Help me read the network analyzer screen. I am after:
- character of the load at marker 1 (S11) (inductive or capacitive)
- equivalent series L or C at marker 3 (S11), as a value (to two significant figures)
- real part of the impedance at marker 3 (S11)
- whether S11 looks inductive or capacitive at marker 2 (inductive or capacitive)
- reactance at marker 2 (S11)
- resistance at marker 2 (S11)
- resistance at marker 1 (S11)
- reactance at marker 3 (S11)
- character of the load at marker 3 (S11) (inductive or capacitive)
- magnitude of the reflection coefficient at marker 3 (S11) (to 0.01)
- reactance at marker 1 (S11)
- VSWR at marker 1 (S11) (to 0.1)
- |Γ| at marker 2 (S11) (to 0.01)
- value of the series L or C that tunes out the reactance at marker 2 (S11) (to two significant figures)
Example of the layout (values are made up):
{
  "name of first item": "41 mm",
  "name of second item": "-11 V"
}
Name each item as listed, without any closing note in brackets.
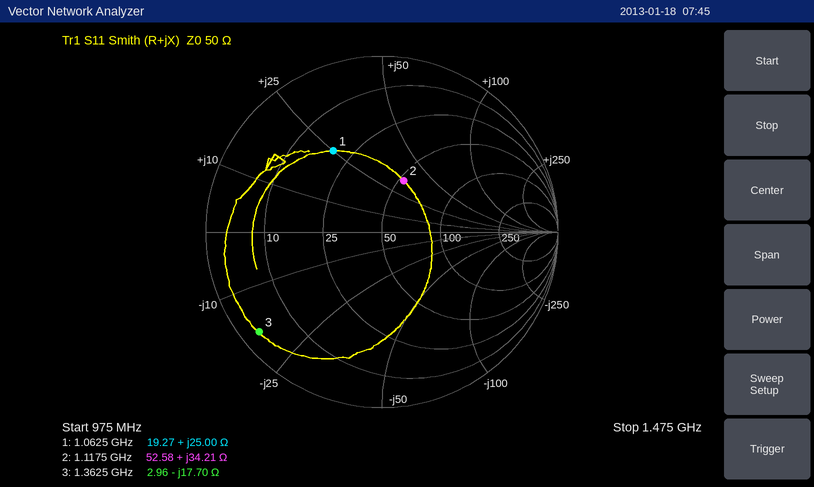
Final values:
{
  "character of the load at marker 1 (S11)": "inductive",
  "equivalent series L or C at marker 3 (S11), as a value": "6.6 pF",
  "real part of the impedance at marker 3": "2.96 Ω",
  "whether S11 looks inductive or capacitive at marker 2": "inductive",
  "reactance at marker 2": "+34.21 Ω",
  "resistance at marker 2": "52.58 Ω",
  "resistance at marker 1": "19.27 Ω",
  "reactance at marker 3": "-17.70 Ω",
  "character of the load at marker 3 (S11)": "capacitive",
  "magnitude of the reflection coefficient at marker 3 (S11)": "0.90",
  "reactance at marker 1": "+25.00 Ω",
  "VSWR at marker 1 (S11)": "3.3",
  "|Γ| at marker 2 (S11)": "0.32",
  "value of the series L or C that tunes out the reactance at marker 2 (S11)": "4.2 pF"
}
